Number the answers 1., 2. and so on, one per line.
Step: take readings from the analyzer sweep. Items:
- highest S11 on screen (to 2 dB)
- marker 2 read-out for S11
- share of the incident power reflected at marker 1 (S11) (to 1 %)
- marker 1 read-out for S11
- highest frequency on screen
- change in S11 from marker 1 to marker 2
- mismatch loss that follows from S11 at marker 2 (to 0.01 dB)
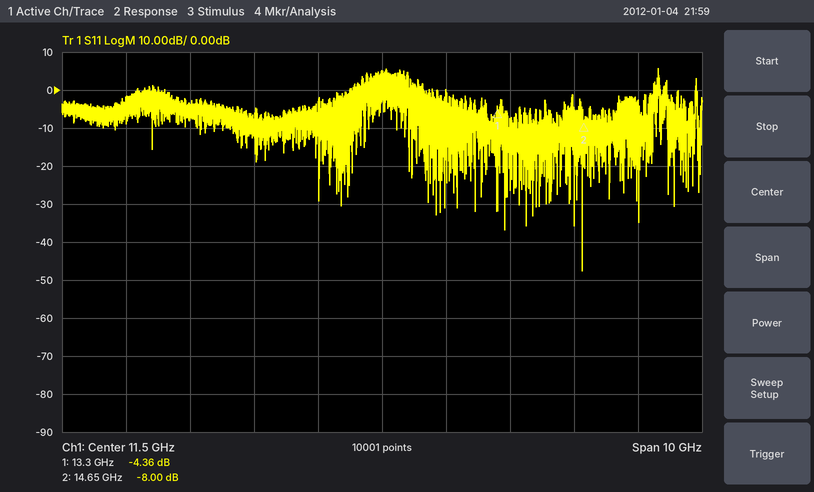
1. 6 dB
2. -8.00 dB
3. 37 %
4. -4.36 dB
5. 16.5 GHz
6. -3.64 dB
7. 0.75 dB
